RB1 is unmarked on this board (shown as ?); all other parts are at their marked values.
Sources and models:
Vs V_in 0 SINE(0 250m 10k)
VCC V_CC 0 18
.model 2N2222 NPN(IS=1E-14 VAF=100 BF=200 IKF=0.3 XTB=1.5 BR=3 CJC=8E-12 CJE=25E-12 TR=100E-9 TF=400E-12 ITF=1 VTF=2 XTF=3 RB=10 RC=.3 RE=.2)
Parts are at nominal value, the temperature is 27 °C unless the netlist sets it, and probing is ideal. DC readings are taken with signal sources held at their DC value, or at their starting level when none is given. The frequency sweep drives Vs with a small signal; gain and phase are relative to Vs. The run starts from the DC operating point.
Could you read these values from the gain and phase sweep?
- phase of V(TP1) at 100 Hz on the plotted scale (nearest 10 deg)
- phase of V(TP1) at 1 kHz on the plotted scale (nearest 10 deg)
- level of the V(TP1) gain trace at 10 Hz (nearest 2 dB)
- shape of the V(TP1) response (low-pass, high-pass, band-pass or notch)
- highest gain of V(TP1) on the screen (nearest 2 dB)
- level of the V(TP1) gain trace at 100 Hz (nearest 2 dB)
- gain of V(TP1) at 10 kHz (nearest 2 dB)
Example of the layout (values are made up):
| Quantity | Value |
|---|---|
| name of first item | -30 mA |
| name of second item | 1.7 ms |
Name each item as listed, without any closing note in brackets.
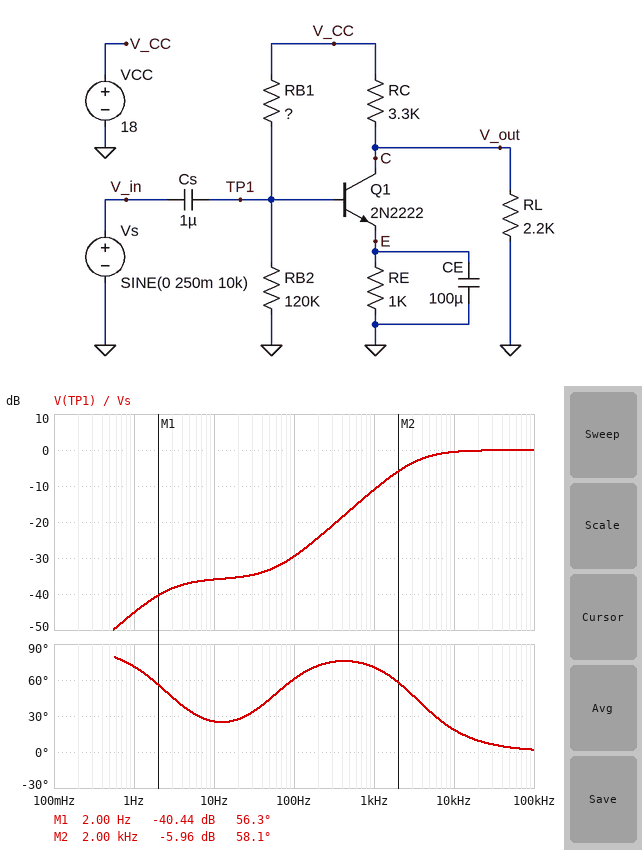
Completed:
| Quantity | Value |
|---|---|
| phase of V(TP1) at 100 Hz on the plotted scale | 60 deg |
| phase of V(TP1) at 1 kHz on the plotted scale | 70 deg |
| level of the V(TP1) gain trace at 10 Hz | -36 dB |
| shape of the V(TP1) response | high-pass |
| highest gain of V(TP1) on the screen | 0 dB |
| level of the V(TP1) gain trace at 100 Hz | -30 dB |
| gain of V(TP1) at 10 kHz | 0 dB |
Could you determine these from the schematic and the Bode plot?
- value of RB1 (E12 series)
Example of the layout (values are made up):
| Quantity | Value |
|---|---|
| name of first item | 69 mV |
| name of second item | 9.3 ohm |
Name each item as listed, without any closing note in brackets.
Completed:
| Quantity | Value |
|---|---|
| value of RB1 | 180 kΩ |
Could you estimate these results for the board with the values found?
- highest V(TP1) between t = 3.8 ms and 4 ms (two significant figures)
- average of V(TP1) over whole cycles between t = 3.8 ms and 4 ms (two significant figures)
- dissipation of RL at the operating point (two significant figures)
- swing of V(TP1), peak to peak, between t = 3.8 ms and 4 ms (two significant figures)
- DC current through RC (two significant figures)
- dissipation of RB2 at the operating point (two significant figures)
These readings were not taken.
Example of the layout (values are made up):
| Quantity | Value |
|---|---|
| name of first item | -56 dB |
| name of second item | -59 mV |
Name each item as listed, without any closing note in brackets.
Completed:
| Quantity | Value |
|---|---|
| highest V(TP1) between t = 3.8 ms and 4 ms | 3.7 V |
| average of V(TP1) over whole cycles between t = 3.8 ms and 4 ms | 3.5 V |
| dissipation of RL at the operating point | 4.6 mW |
| swing of V(TP1), peak to peak, between t = 3.8 ms and 4 ms | 500 mV |
| DC current through RC | 4.5 mA |
| dissipation of RB2 at the operating point | 120 µW |
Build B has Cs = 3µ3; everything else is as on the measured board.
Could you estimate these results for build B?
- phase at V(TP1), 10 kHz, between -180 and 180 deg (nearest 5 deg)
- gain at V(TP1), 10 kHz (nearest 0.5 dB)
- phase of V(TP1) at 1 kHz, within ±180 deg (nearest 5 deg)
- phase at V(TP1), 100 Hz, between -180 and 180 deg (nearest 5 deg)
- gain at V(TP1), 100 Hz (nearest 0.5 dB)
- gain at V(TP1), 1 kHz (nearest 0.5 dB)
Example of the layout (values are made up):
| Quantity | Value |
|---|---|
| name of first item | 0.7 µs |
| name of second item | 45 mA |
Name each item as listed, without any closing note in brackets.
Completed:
| Quantity | Value |
|---|---|
| phase at V(TP1), 10 kHz, between -180 and 180 deg | 5 deg |
| gain at V(TP1), 10 kHz | 0 dB |
| phase of V(TP1) at 1 kHz, within ±180 deg | 45 deg |
| phase at V(TP1), 100 Hz, between -180 and 180 deg | 55 deg |
| gain at V(TP1), 100 Hz | -19.5 dB |
| gain at V(TP1), 1 kHz | -3.5 dB |
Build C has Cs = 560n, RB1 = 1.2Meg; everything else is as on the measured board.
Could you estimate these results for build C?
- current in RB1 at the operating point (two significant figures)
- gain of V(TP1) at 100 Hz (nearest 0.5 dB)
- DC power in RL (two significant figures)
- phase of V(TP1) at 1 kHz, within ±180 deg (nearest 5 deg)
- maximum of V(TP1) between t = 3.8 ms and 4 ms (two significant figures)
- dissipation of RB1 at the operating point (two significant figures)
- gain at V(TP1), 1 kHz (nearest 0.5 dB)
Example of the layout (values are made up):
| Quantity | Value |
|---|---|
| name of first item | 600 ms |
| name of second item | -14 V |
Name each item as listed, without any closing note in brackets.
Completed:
| Quantity | Value |
|---|---|
| current in RB1 at the operating point | 14 µA |
| gain of V(TP1) at 100 Hz | -1.5 dB |
| DC power in RL | 18 mW |
| phase of V(TP1) at 1 kHz, within ±180 deg | 0 deg |
| maximum of V(TP1) between t = 3.8 ms and 4 ms | 1.4 V |
| dissipation of RB1 at the operating point | 230 µW |
| gain at V(TP1), 1 kHz | 0 dB |
